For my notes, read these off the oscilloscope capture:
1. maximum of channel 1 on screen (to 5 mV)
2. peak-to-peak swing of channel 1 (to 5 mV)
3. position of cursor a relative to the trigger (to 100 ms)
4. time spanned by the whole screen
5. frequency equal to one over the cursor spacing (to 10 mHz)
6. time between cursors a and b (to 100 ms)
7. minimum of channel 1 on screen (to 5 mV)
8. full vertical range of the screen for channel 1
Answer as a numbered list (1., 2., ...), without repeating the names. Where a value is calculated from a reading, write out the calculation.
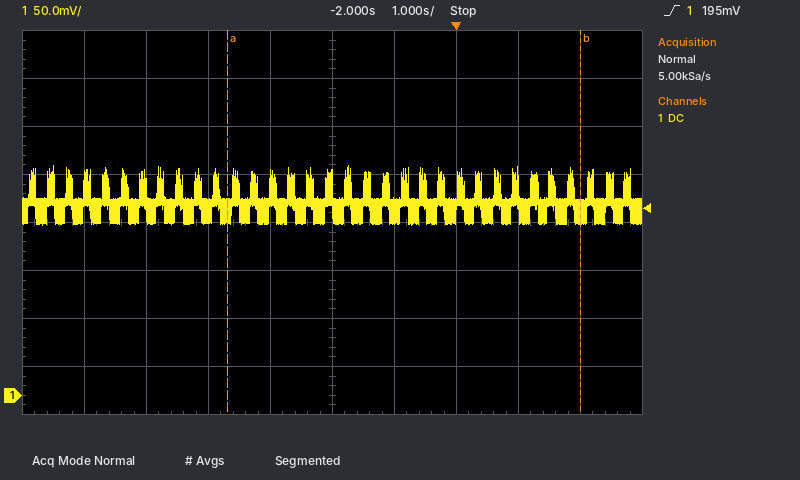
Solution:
1. 240 mV
2. 240 mV − (180 mV) = 60 mV
3. -3.7 s
4. 10 s
5. 1 / 5.7 s ≈ 180 mHz
6. 5.7 s
7. 180 mV
8. 400 mV
